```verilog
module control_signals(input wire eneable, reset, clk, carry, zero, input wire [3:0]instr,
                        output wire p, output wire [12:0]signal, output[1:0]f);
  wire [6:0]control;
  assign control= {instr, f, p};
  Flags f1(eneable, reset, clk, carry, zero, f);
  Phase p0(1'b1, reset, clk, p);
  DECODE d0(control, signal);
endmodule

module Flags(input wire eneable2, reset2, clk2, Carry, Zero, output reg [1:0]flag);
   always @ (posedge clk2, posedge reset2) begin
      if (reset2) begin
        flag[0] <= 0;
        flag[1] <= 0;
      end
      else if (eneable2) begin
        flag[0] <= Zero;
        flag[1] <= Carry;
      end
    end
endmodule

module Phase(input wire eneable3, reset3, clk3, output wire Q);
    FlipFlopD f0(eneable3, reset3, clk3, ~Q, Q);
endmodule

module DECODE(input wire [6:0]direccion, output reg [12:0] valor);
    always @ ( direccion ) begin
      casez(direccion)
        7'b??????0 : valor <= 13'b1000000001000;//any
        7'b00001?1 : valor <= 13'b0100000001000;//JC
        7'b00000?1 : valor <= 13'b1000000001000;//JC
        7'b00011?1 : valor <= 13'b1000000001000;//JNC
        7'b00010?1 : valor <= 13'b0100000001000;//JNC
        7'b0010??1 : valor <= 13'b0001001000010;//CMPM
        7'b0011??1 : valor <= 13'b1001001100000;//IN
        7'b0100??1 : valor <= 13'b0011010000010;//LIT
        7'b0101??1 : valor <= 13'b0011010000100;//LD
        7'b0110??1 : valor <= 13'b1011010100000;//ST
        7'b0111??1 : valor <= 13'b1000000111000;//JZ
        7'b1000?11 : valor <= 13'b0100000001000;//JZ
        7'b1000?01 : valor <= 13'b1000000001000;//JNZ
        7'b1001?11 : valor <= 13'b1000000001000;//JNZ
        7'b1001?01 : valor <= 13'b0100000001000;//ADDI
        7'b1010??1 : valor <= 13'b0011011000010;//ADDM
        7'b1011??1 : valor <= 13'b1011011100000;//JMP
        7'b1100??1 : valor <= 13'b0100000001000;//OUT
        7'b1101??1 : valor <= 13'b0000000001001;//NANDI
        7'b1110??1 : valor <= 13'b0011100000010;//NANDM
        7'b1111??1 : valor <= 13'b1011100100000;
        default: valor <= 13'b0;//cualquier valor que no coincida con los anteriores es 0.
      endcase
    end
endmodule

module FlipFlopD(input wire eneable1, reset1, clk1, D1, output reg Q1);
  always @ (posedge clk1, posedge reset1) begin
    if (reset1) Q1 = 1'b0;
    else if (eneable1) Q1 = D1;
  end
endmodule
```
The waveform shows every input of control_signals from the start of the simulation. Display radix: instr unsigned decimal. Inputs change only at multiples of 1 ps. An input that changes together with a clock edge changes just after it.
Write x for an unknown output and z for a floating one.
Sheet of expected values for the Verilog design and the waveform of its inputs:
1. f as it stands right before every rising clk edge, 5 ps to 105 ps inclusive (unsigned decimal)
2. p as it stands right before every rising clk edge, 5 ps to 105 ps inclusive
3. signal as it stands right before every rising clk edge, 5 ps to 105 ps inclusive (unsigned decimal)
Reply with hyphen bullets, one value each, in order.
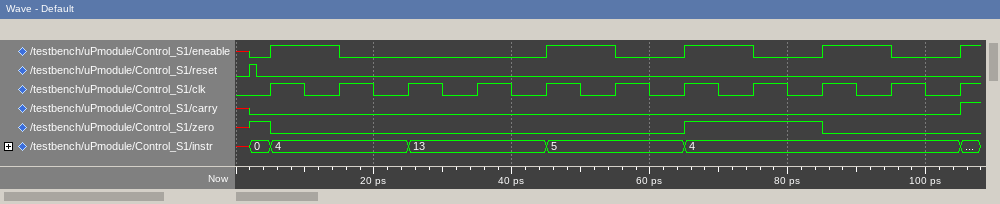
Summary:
- 0, 0, 0, 0, 0, 0, 0, 0, 1, 1, 0
- 0 1 0 1 0 1 0 1 0 1 0
- 4104, 1666, 4104, 9, 4104, 1668, 4104, 1666, 4104, 1666, 4104
